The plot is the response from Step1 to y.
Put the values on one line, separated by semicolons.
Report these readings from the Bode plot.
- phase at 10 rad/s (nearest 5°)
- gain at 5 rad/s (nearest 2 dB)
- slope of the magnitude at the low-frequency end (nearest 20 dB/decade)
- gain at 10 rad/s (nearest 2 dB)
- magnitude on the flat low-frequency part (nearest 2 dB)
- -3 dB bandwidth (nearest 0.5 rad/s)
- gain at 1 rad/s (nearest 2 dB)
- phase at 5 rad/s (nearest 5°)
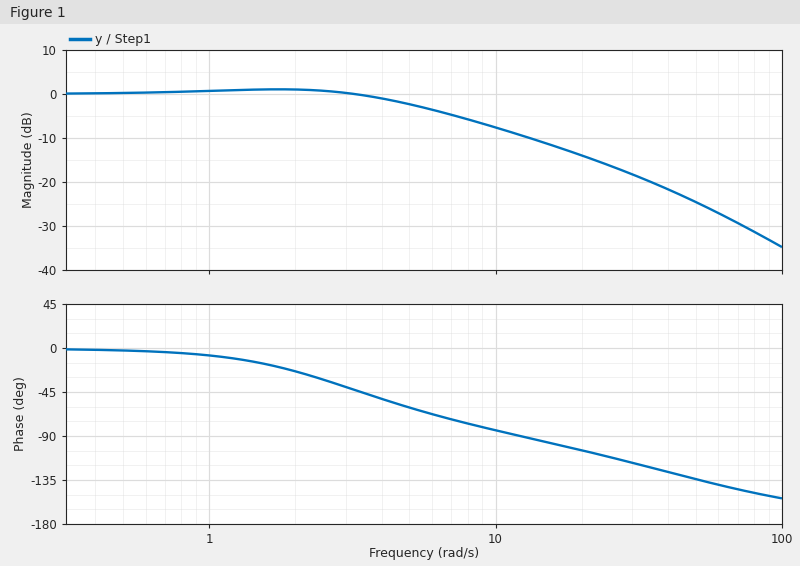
-85°; -2 dB; 0 dB/decade; -8 dB; 0 dB; 5.5 rad/s; 0 dB; -60°
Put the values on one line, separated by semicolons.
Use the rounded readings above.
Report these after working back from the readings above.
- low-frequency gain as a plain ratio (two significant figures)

1.0
